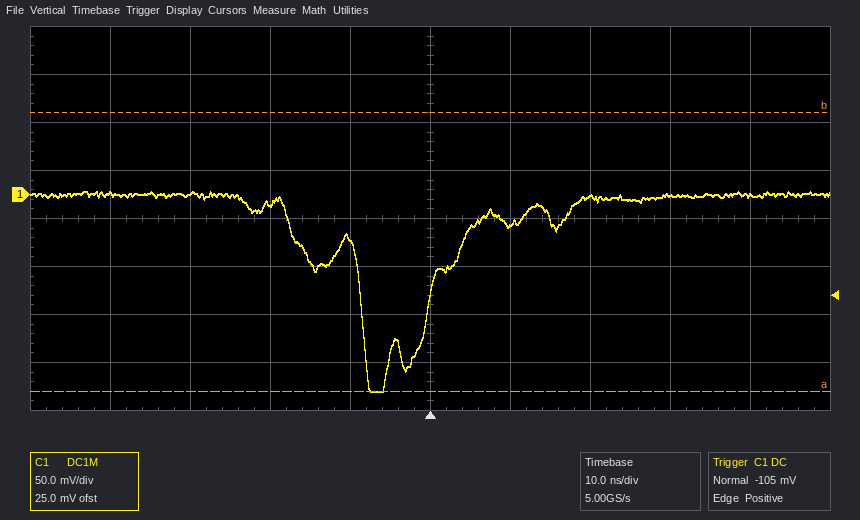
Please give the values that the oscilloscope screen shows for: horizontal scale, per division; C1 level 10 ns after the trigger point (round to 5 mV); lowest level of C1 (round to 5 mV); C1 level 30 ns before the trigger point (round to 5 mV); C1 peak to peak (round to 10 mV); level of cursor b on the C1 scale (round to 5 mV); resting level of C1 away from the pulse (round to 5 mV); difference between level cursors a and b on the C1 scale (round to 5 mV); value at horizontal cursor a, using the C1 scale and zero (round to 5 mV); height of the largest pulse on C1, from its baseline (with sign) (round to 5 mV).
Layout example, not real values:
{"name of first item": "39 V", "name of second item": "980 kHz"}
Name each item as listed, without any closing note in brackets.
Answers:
{"horizontal scale, per division": "10 ns", "C1 level 10 ns after the trigger point": "-30 mV", "lowest level of C1": "-205 mV", "C1 level 30 ns before the trigger point": "0 mV", "C1 peak to peak": "210 mV", "level of cursor b on the C1 scale": "85 mV", "resting level of C1 away from the pulse": "0 mV", "difference between level cursors a and b on the C1 scale": "290 mV", "value at horizontal cursor a, using the C1 scale and zero": "-205 mV", "height of the largest pulse on C1, from its baseline (with sign)": "-205 mV"}
